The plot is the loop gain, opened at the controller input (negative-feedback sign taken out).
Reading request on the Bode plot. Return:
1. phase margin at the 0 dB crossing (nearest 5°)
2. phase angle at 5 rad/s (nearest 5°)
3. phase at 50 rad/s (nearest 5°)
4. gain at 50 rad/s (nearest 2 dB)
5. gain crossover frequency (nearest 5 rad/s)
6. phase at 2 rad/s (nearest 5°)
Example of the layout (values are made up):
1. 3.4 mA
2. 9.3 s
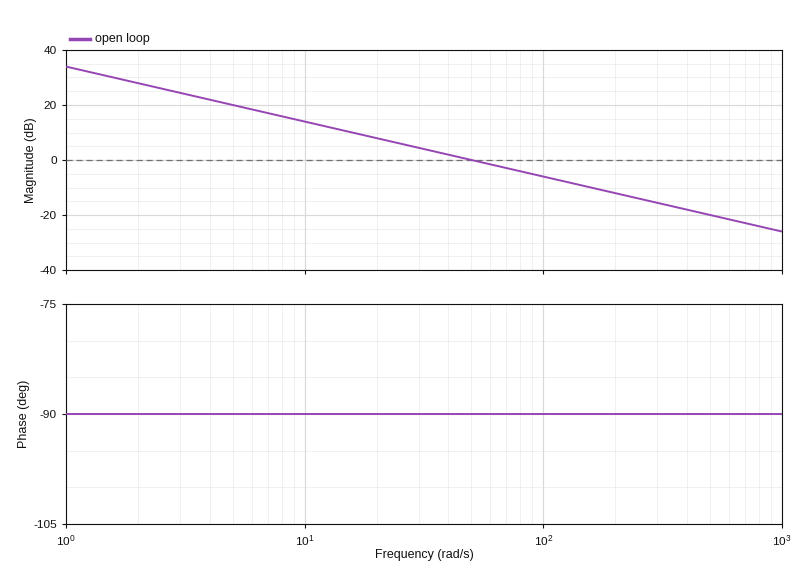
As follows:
1. 90°
2. -90°
3. -90°
4. 0 dB
5. 50 rad/s
6. -90°
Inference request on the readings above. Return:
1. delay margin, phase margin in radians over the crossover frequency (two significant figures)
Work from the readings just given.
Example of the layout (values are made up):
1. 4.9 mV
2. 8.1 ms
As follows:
1. 0.031 s
